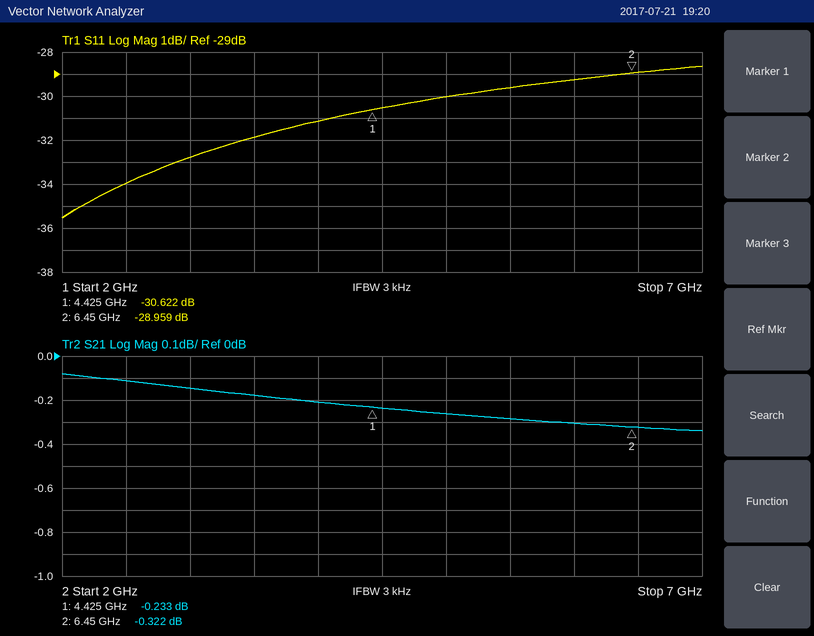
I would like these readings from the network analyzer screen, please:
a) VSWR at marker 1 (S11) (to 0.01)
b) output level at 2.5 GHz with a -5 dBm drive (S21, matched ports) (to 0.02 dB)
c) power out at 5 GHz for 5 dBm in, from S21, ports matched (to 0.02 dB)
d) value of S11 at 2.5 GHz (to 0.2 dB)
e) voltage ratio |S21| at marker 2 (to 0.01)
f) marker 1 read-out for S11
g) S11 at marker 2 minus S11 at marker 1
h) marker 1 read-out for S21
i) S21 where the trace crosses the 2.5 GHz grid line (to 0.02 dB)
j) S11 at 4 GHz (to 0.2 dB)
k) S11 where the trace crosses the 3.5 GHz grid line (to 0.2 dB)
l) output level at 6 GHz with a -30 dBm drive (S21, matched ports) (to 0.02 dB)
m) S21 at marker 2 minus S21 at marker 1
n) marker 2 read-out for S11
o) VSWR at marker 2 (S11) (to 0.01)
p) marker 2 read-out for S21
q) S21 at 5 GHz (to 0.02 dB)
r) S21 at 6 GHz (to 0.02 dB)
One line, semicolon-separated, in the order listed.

1.06; -5.12 dBm; 4.74 dBm; -34.0 dB; 0.96; -30.622 dB; 1.663 dB; -0.233 dB; -0.12 dB; -31.2 dB; -31.8 dB; -30.30 dBm; -0.089 dB; -28.959 dB; 1.07; -0.322 dB; -0.26 dB; -0.30 dB
